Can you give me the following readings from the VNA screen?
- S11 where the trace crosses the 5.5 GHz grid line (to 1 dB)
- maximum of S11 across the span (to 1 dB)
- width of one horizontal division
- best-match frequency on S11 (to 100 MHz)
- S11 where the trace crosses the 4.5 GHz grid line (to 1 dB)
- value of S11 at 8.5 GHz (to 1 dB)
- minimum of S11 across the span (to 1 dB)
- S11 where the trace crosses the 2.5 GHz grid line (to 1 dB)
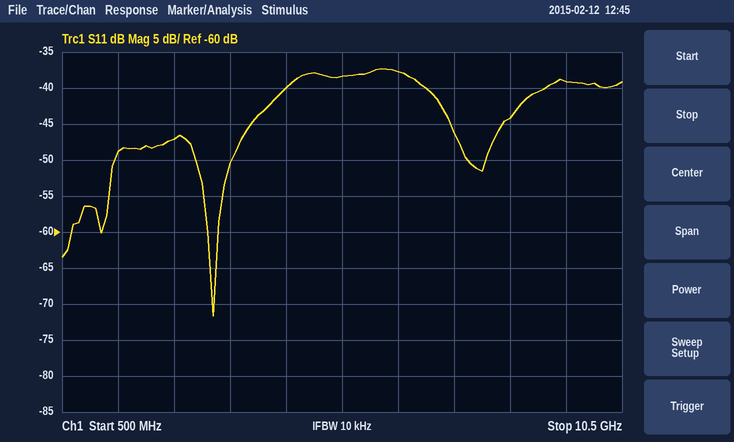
-38 dB
-37 dB
1 GHz
3.2 GHz
-40 dB
-44 dB
-72 dB
-47 dB
